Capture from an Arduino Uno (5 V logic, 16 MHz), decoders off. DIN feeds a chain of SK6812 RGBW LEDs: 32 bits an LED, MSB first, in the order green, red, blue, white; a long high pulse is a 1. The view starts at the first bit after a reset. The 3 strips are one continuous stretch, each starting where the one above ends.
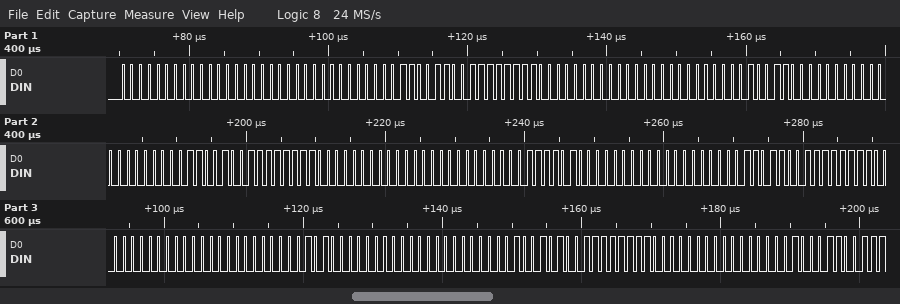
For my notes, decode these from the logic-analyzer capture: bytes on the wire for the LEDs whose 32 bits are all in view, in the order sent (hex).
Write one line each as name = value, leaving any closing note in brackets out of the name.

bytes on the wire for the LEDs whose 32 bits are all in view, in the order sent = 00 00 00 00 CC FF 00 00 00 98 00 00 64 FF 00 00 00 F4 00 00 6C FF 00 00 00 A0 00 00 94 FF 00 00
